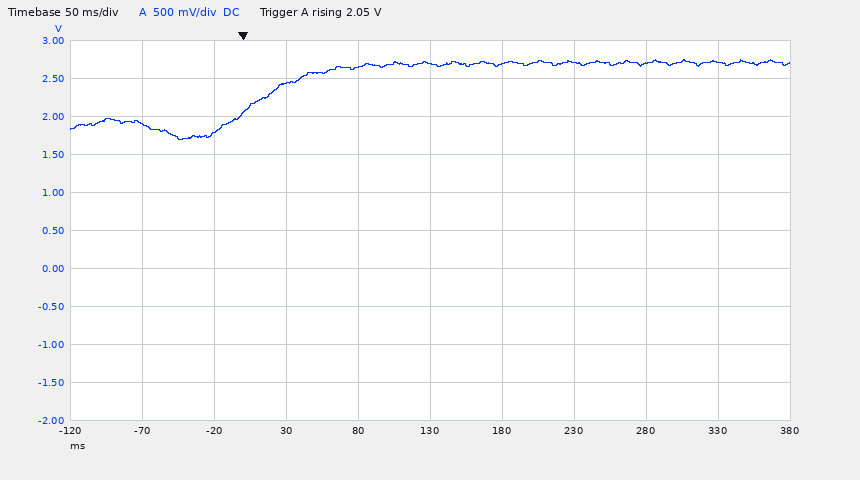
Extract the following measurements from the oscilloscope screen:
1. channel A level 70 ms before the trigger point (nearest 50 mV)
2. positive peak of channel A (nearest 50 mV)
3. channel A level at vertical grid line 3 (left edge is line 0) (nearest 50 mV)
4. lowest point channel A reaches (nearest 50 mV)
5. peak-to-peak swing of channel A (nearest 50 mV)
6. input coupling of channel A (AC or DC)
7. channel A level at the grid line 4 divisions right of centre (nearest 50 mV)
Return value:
1.90 V
2.75 V
2.45 V
1.70 V
1.05 V
DC
2.70 V
